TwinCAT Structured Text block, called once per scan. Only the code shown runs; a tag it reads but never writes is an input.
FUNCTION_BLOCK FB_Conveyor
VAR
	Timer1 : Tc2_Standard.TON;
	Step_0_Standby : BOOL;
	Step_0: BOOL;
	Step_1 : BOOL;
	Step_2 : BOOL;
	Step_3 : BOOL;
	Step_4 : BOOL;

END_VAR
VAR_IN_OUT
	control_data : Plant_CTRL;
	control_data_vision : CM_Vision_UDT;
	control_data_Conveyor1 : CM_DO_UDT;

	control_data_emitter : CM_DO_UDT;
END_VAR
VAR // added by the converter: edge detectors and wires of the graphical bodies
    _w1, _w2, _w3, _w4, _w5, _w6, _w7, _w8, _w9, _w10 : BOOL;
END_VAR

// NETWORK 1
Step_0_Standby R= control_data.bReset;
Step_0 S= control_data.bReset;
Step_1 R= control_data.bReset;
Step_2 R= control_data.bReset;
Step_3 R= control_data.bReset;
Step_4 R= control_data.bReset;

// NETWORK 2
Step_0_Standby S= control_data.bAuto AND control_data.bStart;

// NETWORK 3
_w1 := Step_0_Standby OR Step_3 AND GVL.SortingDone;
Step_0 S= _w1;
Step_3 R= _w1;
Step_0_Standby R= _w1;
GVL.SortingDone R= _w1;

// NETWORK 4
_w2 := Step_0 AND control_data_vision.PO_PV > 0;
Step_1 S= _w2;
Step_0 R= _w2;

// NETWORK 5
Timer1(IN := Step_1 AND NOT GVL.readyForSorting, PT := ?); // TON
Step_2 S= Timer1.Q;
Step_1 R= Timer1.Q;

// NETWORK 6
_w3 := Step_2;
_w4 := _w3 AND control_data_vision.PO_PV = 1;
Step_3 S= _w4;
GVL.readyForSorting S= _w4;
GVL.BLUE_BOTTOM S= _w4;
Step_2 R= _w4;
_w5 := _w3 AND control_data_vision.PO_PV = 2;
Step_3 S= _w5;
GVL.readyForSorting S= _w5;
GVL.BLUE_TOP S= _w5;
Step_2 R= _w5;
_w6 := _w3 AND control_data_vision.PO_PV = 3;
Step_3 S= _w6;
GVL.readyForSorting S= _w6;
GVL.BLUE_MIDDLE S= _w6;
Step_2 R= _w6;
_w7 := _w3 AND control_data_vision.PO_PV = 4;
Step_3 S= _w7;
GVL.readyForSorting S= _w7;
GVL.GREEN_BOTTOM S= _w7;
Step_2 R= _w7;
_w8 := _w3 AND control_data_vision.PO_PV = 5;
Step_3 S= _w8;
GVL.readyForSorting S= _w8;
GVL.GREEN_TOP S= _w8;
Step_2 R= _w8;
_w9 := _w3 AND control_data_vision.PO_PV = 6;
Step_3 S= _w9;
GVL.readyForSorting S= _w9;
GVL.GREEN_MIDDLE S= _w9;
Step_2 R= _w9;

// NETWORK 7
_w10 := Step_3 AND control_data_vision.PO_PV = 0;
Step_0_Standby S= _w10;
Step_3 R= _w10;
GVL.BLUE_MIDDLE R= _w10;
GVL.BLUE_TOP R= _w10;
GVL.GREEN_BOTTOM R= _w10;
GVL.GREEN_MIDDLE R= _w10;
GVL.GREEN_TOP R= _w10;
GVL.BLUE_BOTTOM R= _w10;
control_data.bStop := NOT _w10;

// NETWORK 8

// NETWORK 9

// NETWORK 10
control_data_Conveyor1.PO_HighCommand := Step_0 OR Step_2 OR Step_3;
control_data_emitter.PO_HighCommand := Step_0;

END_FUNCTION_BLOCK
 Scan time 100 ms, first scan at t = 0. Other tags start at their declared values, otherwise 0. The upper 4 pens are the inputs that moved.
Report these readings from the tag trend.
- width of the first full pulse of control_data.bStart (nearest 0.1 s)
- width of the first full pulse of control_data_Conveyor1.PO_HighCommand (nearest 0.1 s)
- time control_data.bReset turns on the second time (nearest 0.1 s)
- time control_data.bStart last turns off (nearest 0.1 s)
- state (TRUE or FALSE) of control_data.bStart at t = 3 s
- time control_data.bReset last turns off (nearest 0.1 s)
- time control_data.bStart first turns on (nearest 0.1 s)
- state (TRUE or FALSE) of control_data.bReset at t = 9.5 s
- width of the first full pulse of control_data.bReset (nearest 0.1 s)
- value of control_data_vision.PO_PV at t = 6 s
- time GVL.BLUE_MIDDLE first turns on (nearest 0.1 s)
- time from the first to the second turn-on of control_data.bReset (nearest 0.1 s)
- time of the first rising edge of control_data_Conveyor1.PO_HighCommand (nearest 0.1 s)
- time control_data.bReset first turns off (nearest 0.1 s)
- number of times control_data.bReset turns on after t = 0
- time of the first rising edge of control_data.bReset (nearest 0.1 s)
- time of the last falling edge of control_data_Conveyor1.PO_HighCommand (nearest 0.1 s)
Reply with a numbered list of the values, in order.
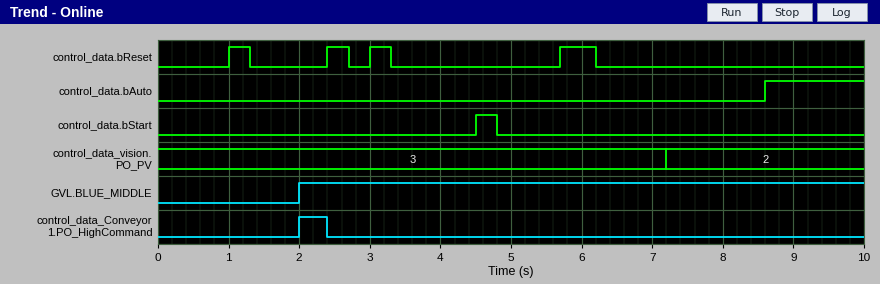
1. 0.3 s
2. 0.4 s
3. 2.4 s
4. 4.8 s
5. FALSE
6. 6.2 s
7. 4.5 s
8. FALSE
9. 0.3 s
10. 3
11. 2.0 s
12. 1.4 s
13. 2.0 s
14. 1.3 s
15. 4
16. 1.0 s
17. 2.4 s
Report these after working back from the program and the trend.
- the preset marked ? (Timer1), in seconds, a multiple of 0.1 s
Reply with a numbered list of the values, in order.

1. 1.0 s
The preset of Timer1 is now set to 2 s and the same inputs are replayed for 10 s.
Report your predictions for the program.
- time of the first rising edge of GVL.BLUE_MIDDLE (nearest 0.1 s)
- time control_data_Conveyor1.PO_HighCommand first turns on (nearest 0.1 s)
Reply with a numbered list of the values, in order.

1. 3.0 s
2. 3.0 s
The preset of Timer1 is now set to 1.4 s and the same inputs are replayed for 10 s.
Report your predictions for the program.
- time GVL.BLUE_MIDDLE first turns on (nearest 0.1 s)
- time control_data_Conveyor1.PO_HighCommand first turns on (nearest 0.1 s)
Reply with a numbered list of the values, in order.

1. 2.4 s
2. 2.4 s
